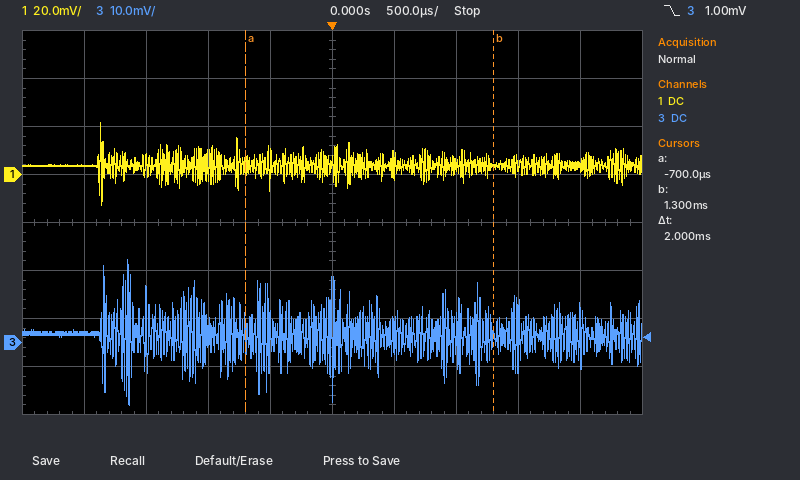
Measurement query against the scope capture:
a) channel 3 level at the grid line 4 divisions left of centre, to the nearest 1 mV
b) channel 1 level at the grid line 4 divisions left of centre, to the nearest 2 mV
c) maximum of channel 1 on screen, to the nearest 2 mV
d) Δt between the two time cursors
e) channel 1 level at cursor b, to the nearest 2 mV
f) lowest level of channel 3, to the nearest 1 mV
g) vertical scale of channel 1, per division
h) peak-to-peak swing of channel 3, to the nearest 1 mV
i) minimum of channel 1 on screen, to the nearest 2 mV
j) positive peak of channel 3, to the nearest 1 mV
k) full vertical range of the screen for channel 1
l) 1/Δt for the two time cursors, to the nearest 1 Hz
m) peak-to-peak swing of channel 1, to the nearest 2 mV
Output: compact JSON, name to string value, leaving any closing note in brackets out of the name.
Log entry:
{"channel 3 level at the grid line 4 divisions left of centre, to the nearest 1 mV": "2 mV", "channel 1 level at the grid line 4 divisions left of centre, to the nearest 2 mV": "4 mV", "maximum of channel 1 on screen, to the nearest 2 mV": "22 mV", "Δt between the two time cursors": "2 ms", "channel 1 level at cursor b, to the nearest 2 mV": "4 mV", "lowest level of channel 3, to the nearest 1 mV": "-13 mV", "vertical scale of channel 1, per division": "20 mV", "peak-to-peak swing of channel 3, to the nearest 1 mV": "30 mV", "minimum of channel 1 on screen, to the nearest 2 mV": "-12 mV", "positive peak of channel 3, to the nearest 1 mV": "17 mV", "full vertical range of the screen for channel 1": "160 mV", "1/Δt for the two time cursors, to the nearest 1 Hz": "500 Hz", "peak-to-peak swing of channel 1, to the nearest 2 mV": "34 mV"}
